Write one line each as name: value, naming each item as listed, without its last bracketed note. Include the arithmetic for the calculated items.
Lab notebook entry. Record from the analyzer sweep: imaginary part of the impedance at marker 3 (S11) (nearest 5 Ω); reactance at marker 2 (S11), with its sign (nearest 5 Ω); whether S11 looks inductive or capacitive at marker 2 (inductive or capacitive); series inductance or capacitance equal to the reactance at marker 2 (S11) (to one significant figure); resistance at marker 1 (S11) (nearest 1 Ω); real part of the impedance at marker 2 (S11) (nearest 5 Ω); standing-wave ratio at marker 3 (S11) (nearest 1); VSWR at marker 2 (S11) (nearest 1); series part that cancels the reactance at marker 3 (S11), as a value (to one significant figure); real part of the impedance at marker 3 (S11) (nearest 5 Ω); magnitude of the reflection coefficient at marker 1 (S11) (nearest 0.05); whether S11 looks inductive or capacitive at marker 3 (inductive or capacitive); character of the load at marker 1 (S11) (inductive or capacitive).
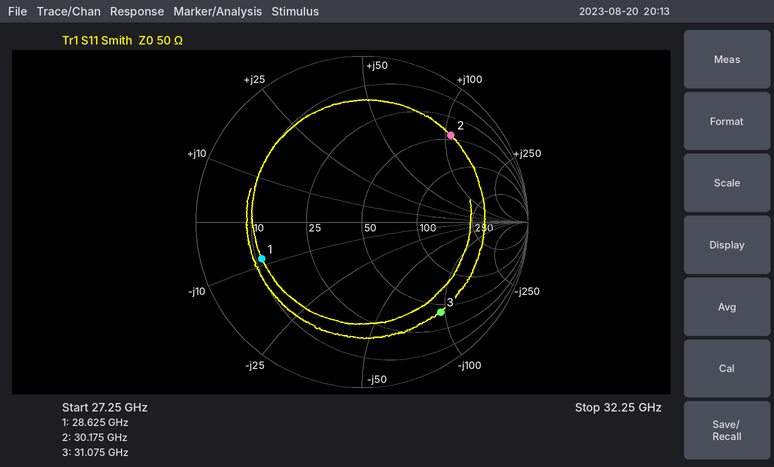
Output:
imaginary part of the impedance at marker 3 (S11): -95 Ω
reactance at marker 2 (S11), with its sign: +105 Ω
whether S11 looks inductive or capacitive at marker 2: inductive
series inductance or capacitance equal to the reactance at marker 2 (S11): L = 105 Ω/(2π × 30.175 GHz) ≈ 554 pH, so 600 pH to one significant figure
resistance at marker 1 (S11): 11 Ω
real part of the impedance at marker 2 (S11): 45 Ω
standing-wave ratio at marker 3 (S11): 6
VSWR at marker 2 (S11): 7
series part that cancels the reactance at marker 3 (S11), as a value: L = 95 Ω/(2π × 31.075 GHz) ≈ 487 pH, so 500 pH to one significant figure
real part of the impedance at marker 3 (S11): 40 Ω
magnitude of the reflection coefficient at marker 1 (S11): 0.65
whether S11 looks inductive or capacitive at marker 3: capacitive
character of the load at marker 1 (S11): capacitive
